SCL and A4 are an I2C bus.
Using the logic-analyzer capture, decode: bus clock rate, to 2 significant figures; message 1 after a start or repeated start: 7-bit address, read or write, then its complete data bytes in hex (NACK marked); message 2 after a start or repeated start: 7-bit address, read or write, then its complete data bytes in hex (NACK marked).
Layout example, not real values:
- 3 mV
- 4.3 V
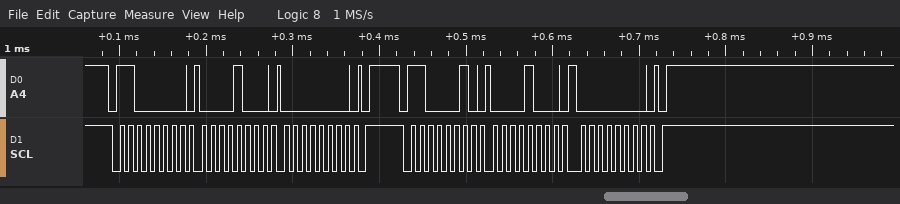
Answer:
- 100 kHz
- 0x60 write: 08 00
- 0x61 write: 08 00
